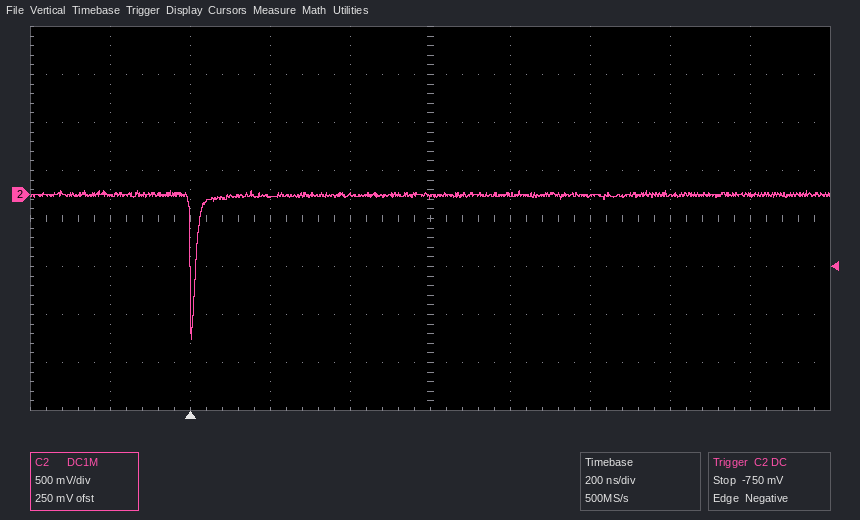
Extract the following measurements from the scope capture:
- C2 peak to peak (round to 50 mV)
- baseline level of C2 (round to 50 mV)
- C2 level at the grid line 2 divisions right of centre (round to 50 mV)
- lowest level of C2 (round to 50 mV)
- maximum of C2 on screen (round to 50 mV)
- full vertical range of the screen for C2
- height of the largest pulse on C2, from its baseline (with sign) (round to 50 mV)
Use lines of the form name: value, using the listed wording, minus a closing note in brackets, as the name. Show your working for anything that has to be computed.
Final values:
C2 peak to peak: 50 mV − (-1.50 V) = 1.55 V
baseline level of C2: 0 mV
C2 level at the grid line 2 divisions right of centre: 0 mV
lowest level of C2: -1.50 V
maximum of C2 on screen: 50 mV
full vertical range of the screen for C2: 4 V
height of the largest pulse on C2, from its baseline (with sign): -1.50 V − (0 mV) = -1.50 V
